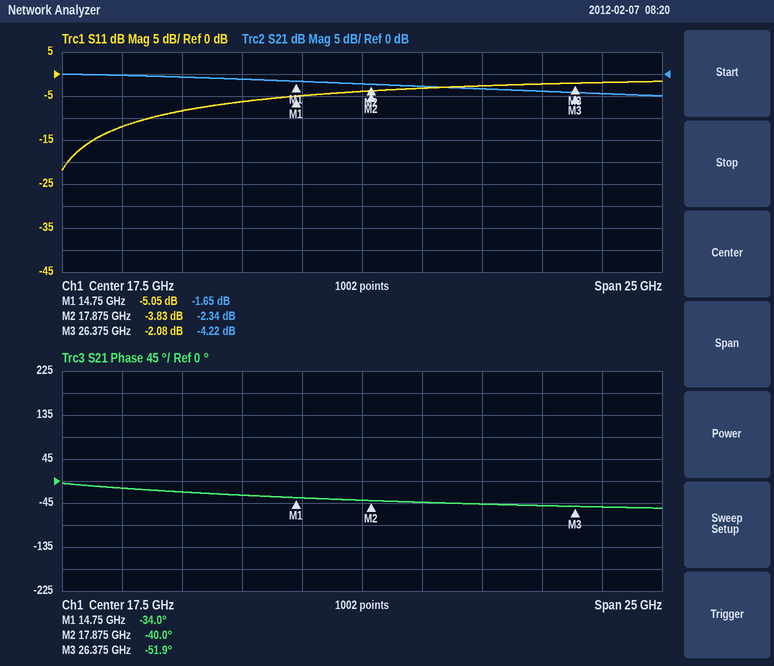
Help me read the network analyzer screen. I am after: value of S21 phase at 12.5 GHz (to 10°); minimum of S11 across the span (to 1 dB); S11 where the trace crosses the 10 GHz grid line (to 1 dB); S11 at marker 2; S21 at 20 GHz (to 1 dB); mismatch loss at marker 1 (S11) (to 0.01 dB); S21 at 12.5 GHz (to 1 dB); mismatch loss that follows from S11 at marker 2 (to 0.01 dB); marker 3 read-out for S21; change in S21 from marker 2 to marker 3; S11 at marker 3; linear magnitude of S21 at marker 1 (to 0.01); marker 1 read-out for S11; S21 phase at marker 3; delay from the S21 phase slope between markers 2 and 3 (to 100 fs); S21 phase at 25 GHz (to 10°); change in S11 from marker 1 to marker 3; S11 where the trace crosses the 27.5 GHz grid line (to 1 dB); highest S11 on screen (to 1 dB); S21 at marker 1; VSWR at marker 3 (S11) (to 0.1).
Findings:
-30°
-22 dB
-8 dB
-3.83 dB
-3 dB
1.63 dB
-1 dB
2.32 dB
-4.22 dB
-1.88 dB
-2.08 dB
0.83
-5.05 dB
-51.9°
3.9 ps
-50°
2.97 dB
-2 dB
-2 dB
-1.65 dB
8.4
